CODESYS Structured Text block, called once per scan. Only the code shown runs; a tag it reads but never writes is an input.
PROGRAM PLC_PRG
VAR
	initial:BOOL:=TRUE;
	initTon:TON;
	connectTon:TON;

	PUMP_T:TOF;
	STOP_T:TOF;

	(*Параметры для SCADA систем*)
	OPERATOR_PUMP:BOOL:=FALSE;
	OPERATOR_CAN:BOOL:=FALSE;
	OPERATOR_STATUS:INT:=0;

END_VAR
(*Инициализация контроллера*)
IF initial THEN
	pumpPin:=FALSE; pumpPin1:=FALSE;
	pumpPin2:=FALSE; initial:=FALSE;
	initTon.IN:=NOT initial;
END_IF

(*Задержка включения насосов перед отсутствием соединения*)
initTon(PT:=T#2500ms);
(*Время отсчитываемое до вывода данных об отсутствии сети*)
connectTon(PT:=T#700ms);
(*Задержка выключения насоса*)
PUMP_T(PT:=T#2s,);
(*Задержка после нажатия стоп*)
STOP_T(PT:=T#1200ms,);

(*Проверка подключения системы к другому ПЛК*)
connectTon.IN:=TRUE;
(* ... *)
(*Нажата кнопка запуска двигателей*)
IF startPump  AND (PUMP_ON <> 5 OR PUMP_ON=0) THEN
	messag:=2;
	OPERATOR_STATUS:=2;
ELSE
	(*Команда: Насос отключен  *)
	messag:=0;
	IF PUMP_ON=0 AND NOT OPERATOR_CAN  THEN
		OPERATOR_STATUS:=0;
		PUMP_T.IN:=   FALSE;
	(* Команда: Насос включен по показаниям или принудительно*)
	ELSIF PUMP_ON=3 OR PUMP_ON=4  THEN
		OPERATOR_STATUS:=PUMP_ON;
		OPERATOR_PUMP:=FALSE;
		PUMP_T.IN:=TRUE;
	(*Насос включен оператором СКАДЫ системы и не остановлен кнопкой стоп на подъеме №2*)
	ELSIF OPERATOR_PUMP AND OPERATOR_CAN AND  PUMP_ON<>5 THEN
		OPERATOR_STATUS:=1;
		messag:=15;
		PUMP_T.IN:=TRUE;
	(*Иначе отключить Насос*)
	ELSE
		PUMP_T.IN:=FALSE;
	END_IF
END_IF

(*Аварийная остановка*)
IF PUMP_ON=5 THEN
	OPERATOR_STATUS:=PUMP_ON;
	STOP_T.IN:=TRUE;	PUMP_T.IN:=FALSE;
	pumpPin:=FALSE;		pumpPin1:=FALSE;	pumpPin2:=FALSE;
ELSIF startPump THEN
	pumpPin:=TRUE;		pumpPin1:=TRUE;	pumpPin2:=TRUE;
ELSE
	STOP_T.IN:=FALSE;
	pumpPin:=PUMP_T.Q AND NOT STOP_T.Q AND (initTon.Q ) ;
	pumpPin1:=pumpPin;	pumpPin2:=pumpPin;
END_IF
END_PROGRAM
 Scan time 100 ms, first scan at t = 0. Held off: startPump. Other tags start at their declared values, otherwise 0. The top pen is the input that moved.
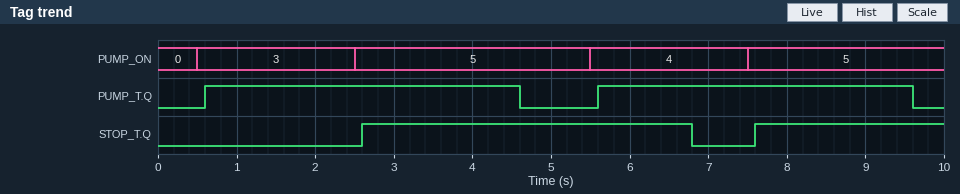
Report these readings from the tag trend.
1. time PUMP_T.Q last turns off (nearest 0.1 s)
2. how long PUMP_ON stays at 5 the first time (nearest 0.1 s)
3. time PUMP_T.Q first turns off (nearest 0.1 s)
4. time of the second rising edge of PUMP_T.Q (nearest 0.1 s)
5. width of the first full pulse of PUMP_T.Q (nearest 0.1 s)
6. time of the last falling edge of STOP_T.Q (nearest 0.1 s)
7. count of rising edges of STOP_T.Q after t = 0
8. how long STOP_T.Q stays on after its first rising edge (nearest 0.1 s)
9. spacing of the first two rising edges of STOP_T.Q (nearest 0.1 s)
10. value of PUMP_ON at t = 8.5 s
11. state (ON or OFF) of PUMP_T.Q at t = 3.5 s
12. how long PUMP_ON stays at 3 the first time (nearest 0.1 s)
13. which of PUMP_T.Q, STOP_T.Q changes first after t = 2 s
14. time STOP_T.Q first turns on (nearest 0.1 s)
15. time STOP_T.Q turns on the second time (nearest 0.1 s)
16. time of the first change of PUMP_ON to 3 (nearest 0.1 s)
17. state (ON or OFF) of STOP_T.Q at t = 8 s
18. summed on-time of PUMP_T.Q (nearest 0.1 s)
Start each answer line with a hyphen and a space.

- 9.6 s
- 3.0 s
- 4.6 s
- 5.6 s
- 4.0 s
- 6.8 s
- 2
- 4.2 s
- 5.0 s
- 5
- ON
- 2.0 s
- STOP_T.Q
- 2.6 s
- 7.6 s
- 0.5 s
- ON
- 8.0 s
